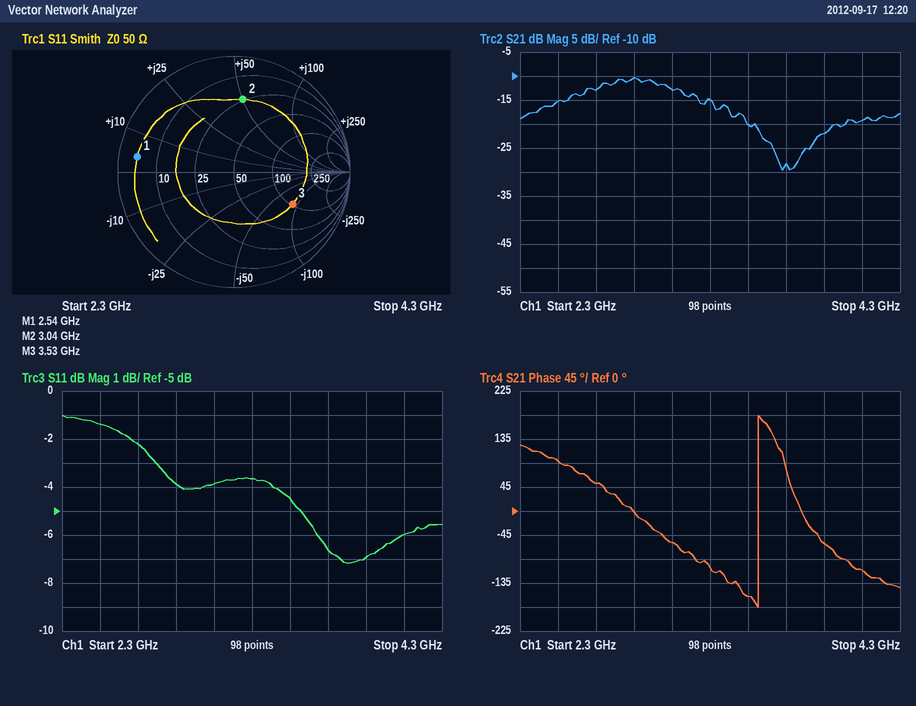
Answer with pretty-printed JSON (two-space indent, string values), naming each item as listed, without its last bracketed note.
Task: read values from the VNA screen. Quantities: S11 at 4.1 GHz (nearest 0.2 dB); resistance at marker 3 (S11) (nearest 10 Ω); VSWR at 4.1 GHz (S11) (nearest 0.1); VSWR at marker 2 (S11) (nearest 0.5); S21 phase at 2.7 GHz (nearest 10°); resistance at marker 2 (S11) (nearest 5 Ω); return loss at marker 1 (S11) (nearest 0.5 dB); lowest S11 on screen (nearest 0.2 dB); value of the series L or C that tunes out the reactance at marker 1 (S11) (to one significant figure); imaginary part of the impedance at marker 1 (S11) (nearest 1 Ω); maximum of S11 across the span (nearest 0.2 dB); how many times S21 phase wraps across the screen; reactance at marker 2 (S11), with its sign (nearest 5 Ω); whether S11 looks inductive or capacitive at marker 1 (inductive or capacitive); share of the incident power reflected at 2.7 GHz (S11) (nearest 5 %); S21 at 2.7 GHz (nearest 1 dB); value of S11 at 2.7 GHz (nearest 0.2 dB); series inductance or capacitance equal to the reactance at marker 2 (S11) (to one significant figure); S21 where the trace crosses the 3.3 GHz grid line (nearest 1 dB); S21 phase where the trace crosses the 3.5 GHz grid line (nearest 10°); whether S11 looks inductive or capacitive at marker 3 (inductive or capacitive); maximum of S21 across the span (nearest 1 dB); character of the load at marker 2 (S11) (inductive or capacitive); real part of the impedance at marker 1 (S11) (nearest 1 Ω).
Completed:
{
  "S11 at 4.1 GHz": "-6.0 dB",
  "resistance at marker 3 (S11)": "100 Ω",
  "VSWR at 4.1 GHz (S11)": "3.0",
  "VSWR at marker 2 (S11)": "4.5",
  "S21 phase at 2.7 GHz": "50°",
  "resistance at marker 2 (S11)": "25 Ω",
  "return loss at marker 1 (S11)": "1.5 dB",
  "lowest S11 on screen": "-7.2 dB",
  "value of the series L or C that tunes out the reactance at marker 1 (S11)": "20 pF",
  "imaginary part of the impedance at marker 1 (S11)": "+4 Ω",
  "maximum of S11 across the span": "-1.0 dB",
  "how many times S21 phase wraps across the screen": "1",
  "reactance at marker 2 (S11), with its sign": "+50 Ω",
  "whether S11 looks inductive or capacitive at marker 1": "inductive",
  "share of the incident power reflected at 2.7 GHz (S11)": "60 %",
  "S21 at 2.7 GHz": "-13 dB",
  "value of S11 at 2.7 GHz": "-2.2 dB",
  "series inductance or capacitance equal to the reactance at marker 2 (S11)": "3 nH",
  "S21 where the trace crosses the 3.3 GHz grid line": "-15 dB",
  "S21 phase where the trace crosses the 3.5 GHz grid line": "-160°",
  "whether S11 looks inductive or capacitive at marker 3": "capacitive",
  "maximum of S21 across the span": "-10 dB",
  "character of the load at marker 2 (S11)": "inductive",
  "real part of the impedance at marker 1 (S11)": "4 Ω"
}
